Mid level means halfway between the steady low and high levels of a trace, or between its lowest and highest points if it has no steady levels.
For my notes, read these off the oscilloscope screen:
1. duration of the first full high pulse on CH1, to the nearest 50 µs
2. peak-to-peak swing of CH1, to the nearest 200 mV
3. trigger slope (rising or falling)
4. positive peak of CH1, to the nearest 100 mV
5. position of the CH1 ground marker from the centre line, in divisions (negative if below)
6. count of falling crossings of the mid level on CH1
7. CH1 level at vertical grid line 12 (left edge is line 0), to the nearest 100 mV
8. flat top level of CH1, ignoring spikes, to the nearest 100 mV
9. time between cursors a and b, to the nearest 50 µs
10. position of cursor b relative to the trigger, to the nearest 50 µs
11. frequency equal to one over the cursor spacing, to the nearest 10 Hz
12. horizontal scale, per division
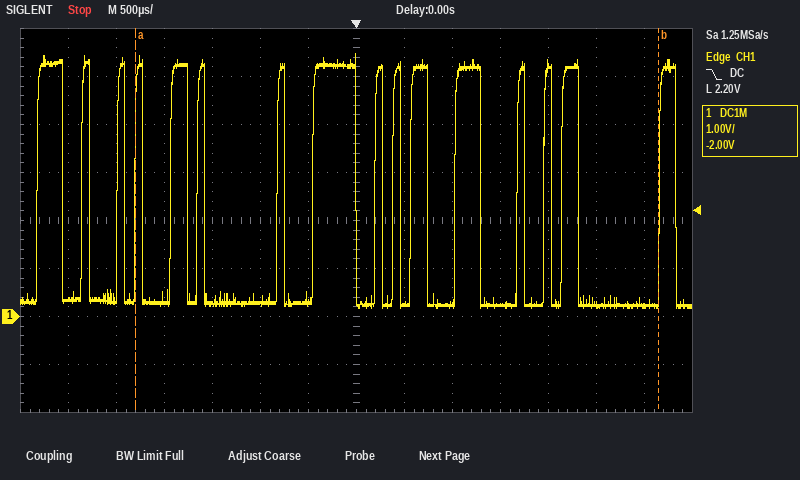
250 µs
5.4 V
falling
5.5 V
-2.0 div
16
200 mV
5.2 V
5.45 ms
+3.15 ms
180 Hz
500 µs
